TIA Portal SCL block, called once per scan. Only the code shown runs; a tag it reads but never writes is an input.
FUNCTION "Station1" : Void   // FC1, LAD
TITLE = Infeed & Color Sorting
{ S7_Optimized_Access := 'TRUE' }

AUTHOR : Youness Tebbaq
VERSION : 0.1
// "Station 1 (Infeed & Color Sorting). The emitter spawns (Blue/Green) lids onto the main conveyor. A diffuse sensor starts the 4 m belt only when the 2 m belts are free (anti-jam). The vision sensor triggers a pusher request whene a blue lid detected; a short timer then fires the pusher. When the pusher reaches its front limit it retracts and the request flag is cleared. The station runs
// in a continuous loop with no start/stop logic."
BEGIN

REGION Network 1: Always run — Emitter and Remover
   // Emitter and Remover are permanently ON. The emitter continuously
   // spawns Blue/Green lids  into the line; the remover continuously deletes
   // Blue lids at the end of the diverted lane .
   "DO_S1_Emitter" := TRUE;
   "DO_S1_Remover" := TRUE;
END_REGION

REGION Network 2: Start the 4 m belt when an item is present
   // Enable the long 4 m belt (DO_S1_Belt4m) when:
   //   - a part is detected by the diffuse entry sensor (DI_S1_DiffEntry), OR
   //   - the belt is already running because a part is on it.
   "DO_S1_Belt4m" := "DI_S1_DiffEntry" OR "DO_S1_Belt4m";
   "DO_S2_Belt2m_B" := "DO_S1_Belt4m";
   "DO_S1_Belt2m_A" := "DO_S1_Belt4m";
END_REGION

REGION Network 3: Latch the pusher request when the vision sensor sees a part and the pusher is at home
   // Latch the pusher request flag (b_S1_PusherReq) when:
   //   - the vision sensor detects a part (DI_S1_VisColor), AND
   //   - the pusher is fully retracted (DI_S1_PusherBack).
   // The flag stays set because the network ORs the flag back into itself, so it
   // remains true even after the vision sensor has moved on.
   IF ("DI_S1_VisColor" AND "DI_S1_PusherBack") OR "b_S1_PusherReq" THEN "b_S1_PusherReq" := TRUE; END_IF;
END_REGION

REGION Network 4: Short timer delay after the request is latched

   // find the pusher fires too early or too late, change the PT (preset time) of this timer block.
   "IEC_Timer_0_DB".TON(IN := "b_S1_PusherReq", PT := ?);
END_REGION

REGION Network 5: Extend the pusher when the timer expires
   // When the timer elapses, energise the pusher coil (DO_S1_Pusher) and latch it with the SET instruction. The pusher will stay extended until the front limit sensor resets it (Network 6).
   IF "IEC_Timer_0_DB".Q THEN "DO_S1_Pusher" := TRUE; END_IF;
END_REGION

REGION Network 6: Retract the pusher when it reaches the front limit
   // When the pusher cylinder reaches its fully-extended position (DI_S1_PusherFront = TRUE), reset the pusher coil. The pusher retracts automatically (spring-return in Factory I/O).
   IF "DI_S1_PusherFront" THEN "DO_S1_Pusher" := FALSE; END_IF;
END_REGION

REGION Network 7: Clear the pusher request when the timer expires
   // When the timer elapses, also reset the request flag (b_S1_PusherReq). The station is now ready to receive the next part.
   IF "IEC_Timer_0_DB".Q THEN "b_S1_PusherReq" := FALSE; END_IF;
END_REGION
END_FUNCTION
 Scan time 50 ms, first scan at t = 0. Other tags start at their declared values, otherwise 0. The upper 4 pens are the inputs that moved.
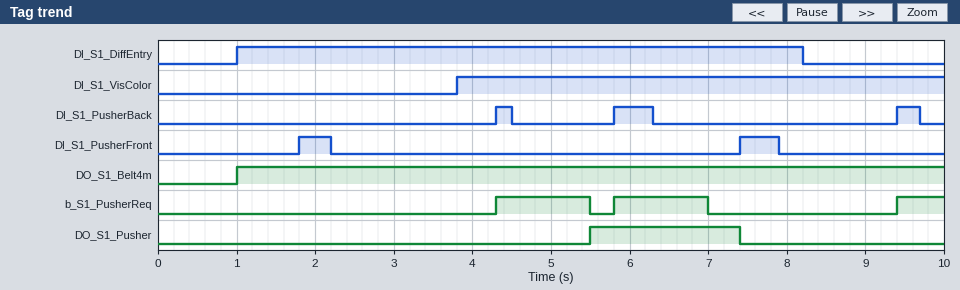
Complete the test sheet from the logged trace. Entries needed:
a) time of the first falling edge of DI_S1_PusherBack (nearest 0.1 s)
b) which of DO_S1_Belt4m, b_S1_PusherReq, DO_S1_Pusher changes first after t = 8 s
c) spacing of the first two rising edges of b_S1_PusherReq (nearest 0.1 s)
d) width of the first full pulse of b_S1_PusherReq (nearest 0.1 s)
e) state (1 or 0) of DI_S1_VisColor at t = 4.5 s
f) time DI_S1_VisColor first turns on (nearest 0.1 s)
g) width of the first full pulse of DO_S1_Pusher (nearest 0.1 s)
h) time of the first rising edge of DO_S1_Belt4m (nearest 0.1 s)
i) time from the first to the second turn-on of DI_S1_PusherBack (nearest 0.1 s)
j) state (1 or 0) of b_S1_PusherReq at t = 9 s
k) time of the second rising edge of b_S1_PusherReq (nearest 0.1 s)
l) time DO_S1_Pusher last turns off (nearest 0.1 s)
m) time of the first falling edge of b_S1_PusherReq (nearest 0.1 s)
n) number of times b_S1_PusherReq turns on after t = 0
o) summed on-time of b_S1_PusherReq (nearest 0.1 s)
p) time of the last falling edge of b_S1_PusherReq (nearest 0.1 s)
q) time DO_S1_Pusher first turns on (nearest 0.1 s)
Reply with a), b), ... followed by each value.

a) 4.5 s
b) b_S1_PusherReq
c) 1.5 s
d) 1.2 s
e) 1
f) 3.8 s
g) 1.9 s
h) 1.0 s
i) 1.5 s
j) 0
k) 5.8 s
l) 7.4 s
m) 5.5 s
n) 3
o) 3.0 s
p) 7.0 s
q) 5.5 s
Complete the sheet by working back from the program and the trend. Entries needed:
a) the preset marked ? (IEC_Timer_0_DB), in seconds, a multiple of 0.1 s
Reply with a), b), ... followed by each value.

a) 1.2 s
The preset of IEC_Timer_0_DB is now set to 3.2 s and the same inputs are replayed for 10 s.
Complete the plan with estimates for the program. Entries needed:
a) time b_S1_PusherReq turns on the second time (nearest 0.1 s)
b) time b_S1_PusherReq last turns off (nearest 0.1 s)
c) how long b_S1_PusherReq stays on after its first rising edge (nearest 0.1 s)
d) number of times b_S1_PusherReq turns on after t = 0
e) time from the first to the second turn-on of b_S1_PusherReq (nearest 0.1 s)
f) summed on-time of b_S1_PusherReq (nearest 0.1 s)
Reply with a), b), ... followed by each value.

a) 9.4 s
b) 7.5 s
c) 3.2 s
d) 2
e) 5.1 s
f) 3.8 s
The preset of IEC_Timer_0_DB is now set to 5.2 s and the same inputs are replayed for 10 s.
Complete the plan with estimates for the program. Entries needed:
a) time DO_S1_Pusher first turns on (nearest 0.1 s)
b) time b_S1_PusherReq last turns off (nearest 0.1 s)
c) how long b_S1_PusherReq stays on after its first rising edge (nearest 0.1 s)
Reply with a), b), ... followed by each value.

a) 9.5 s
b) 9.5 s
c) 5.2 s
